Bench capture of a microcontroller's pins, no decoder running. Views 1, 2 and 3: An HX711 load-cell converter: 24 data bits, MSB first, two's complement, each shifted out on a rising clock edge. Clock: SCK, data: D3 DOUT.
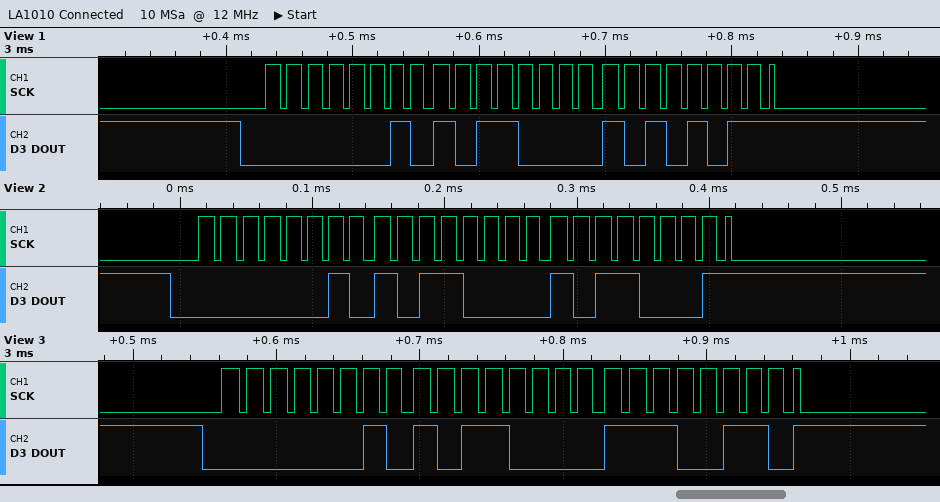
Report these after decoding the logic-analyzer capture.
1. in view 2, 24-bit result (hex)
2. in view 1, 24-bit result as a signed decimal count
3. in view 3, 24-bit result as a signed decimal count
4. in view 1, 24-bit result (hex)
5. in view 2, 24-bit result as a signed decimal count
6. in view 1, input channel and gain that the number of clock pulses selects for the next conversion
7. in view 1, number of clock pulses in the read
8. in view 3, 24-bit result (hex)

0x02B0B1
176299
176358
0x02B0AB
176305
channel A, gain 128
25
0x02B0E6
